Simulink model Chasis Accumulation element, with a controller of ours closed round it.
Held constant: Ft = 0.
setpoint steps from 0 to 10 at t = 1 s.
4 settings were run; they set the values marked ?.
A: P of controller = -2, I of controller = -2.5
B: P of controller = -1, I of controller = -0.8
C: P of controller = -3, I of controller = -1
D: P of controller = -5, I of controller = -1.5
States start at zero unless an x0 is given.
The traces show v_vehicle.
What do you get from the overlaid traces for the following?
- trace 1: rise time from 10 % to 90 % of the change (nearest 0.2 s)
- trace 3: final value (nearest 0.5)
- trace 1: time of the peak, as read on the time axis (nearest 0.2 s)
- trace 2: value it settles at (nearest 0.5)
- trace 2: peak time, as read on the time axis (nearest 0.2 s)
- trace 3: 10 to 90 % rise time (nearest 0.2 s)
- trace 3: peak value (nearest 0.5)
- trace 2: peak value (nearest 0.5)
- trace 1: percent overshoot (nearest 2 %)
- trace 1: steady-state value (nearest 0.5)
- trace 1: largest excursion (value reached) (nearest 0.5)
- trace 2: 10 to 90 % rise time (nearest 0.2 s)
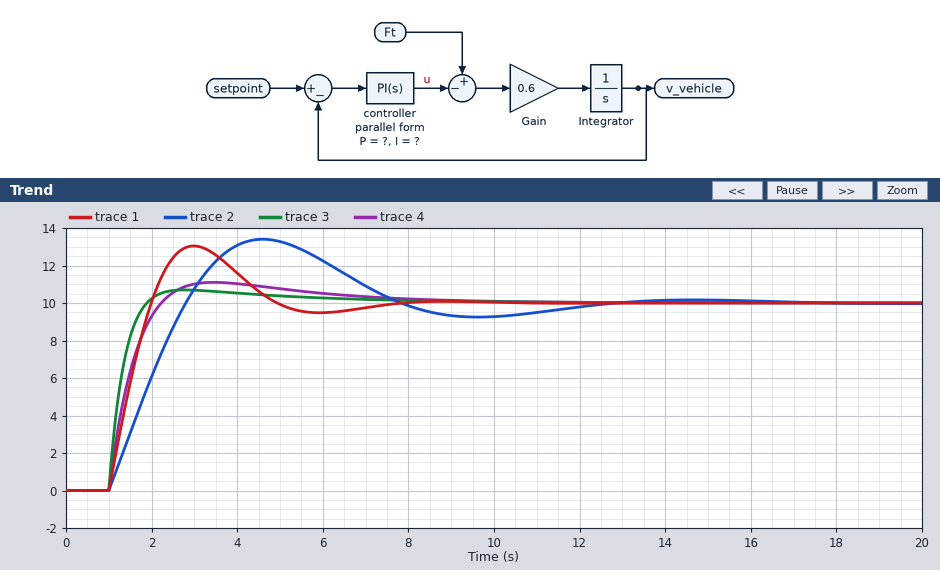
0.8 s
10.0
3.0 s
10.0
4.6 s
0.6 s
10.5
13.5
30 %
10.0
13.0
1.4 s
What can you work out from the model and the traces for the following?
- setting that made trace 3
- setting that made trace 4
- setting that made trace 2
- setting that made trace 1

D
C
B
A
